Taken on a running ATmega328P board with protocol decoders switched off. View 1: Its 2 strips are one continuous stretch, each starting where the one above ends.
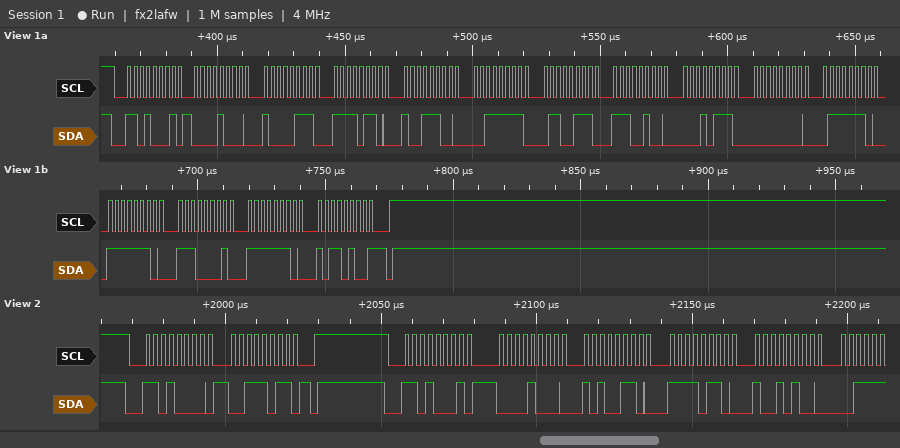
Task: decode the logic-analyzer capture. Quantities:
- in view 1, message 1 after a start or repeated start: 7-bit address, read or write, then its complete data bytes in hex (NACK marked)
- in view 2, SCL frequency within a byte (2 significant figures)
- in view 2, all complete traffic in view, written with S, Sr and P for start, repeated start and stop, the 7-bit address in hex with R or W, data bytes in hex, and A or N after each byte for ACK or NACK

0x68 read: 08 87 F6 9C 3F 67 E4 17 00 7E FE E1 FE B4 NACK
400 kHz
S 68W A 3B A P S 68R A 08 A A6 A F6 A 94 A
